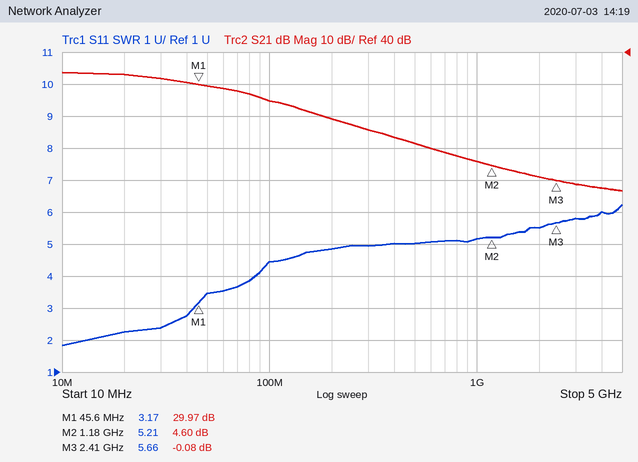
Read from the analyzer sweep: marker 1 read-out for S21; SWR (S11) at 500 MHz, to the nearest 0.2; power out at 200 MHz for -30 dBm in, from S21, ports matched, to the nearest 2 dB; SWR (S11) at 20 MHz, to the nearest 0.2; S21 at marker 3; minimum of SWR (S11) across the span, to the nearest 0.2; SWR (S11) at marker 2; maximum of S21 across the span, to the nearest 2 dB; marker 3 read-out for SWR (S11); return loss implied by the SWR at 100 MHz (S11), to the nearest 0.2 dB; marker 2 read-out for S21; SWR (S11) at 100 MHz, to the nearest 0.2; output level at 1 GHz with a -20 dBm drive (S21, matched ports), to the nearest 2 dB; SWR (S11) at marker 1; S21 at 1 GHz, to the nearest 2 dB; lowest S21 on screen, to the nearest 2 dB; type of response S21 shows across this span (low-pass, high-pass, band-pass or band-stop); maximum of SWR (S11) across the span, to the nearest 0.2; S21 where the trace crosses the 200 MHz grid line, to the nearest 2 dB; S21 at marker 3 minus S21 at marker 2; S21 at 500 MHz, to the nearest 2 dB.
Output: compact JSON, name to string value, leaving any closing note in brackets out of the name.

{"marker 1 read-out for S21": "29.97 dB", "SWR (S11) at 500 MHz, to the nearest 0.2": "5.0", "power out at 200 MHz for -30 dBm in, from S21, ports matched, to the nearest 2 dB": "-10 dBm", "SWR (S11) at 20 MHz, to the nearest 0.2": "2.2", "S21 at marker 3": "-0.08 dB", "minimum of SWR (S11) across the span, to the nearest 0.2": "1.8", "SWR (S11) at marker 2": "5.21", "maximum of S21 across the span, to the nearest 2 dB": "34 dB", "marker 3 read-out for SWR": "5.66", "return loss implied by the SWR at 100 MHz (S11), to the nearest 0.2 dB": "4.0 dB", "marker 2 read-out for S21": "4.60 dB", "SWR (S11) at 100 MHz, to the nearest 0.2": "4.4", "output level at 1 GHz with a -20 dBm drive (S21, matched ports), to the nearest 2 dB": "-14 dBm", "SWR (S11) at marker 1": "3.17", "S21 at 1 GHz, to the nearest 2 dB": "6 dB", "lowest S21 on screen, to the nearest 2 dB": "-4 dB", "type of response S21 shows across this span": "low-pass", "maximum of SWR (S11) across the span, to the nearest 0.2": "6.2", "S21 where the trace crosses the 200 MHz grid line, to the nearest 2 dB": "20 dB", "S21 at marker 3 minus S21 at marker 2": "-4.68 dB", "S21 at 500 MHz, to the nearest 2 dB": "12 dB"}
